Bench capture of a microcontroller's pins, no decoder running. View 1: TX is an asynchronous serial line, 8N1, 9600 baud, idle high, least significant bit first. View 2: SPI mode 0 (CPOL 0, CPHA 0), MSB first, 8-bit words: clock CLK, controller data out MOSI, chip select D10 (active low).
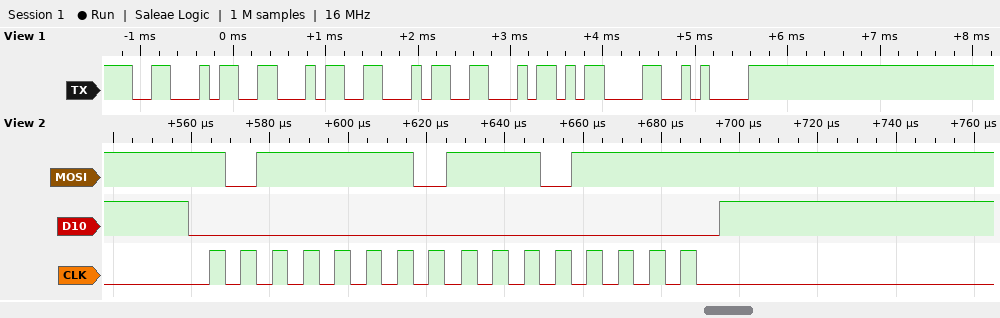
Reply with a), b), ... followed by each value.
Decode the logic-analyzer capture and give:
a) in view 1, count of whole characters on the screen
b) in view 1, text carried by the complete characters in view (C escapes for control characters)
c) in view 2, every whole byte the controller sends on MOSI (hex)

a) 6
b) "FFFF\r\n"
c) 0xBE 0xEF
